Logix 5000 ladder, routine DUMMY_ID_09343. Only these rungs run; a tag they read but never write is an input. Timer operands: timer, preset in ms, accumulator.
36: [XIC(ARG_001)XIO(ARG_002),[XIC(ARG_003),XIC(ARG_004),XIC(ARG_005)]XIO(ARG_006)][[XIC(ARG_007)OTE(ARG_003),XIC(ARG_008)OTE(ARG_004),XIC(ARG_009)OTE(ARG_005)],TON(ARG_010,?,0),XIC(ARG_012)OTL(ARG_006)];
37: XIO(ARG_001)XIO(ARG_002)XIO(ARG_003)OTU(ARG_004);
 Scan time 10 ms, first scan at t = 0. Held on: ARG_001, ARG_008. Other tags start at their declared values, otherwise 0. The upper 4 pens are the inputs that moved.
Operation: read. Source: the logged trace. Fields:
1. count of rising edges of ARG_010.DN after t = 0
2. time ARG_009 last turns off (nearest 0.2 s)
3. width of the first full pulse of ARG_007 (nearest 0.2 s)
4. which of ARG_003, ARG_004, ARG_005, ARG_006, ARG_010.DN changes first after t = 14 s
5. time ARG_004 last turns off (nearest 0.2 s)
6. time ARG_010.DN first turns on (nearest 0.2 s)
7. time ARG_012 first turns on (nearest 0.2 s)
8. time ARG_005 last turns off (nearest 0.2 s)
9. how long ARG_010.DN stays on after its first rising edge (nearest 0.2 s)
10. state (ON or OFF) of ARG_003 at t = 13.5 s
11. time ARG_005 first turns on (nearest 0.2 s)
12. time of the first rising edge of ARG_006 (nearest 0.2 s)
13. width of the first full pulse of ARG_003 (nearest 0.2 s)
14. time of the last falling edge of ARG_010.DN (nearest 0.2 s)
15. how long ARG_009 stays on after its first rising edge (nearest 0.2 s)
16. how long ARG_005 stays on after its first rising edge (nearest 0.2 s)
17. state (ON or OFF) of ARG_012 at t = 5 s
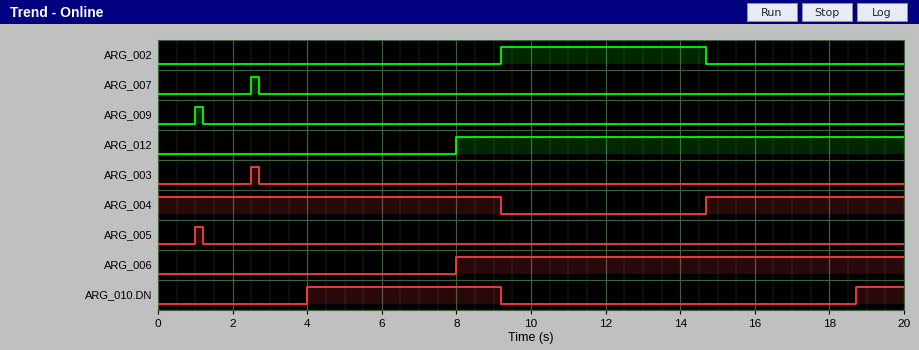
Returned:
2
1.2 s
0.2 s
ARG_004
9.2 s
4.0 s
8.0 s
1.2 s
5.2 s
OFF
1.0 s
8.0 s
0.2 s
9.2 s
0.2 s
0.2 s
OFF
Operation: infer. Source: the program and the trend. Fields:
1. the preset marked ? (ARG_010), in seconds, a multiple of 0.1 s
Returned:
4.0 s
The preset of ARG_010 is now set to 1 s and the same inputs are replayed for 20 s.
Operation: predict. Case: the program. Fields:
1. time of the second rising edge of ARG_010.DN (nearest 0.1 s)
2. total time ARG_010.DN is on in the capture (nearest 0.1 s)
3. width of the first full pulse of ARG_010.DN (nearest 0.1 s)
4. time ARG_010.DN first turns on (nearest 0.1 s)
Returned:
15.7 s
12.5 s
8.2 s
1.0 s
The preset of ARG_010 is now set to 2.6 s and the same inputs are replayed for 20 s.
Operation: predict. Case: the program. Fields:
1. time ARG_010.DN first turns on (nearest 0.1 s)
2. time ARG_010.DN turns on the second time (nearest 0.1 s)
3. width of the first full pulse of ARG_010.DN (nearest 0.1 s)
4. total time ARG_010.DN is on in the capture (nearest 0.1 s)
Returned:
2.6 s
17.3 s
6.6 s
9.3 s
